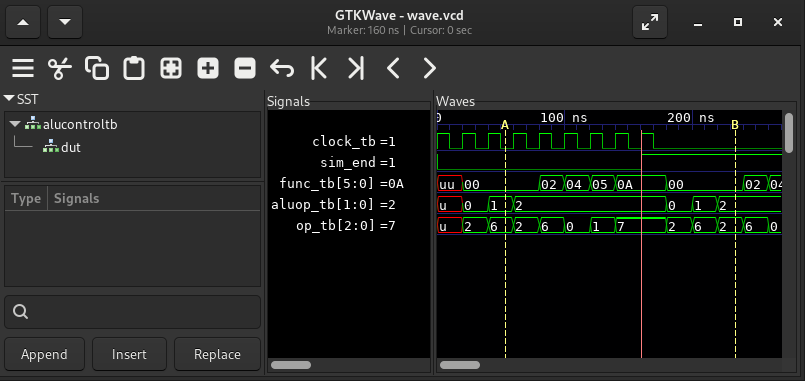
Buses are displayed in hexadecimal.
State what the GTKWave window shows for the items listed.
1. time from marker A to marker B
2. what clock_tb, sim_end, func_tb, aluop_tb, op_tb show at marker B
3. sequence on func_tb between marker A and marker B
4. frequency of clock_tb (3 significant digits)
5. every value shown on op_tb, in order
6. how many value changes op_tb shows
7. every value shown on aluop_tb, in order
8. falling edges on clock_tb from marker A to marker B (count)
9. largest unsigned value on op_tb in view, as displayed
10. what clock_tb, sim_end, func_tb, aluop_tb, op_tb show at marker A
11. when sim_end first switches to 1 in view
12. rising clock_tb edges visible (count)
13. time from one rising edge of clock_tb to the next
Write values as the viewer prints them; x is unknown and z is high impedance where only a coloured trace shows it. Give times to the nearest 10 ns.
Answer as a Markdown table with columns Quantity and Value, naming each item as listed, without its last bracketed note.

| Quantity | Value |
|---|---|
| time from marker A to marker B | 180 ns |
| what clock_tb, sim_end, func_tb, aluop_tb, op_tb show at marker B | clock_tb=0, sim_end=1, func_tb=00, aluop_tb=2, op_tb=2 |
| sequence on func_tb between marker A and marker B | 00, 02, 04, 05, 0A, 00 |
| frequency of clock_tb | 50.0 MHz |
| every value shown on op_tb, in order | u, 2, 6, 2, 6, 0, 1, 7, 2, 6, 2, 6, 0 |
| how many value changes op_tb shows | 12 |
| every value shown on aluop_tb, in order | u, 0, 1, 2, 0, 1, 2 |
| falling edges on clock_tb from marker A to marker B | 6 |
| largest unsigned value on op_tb in view, as displayed | 7 |
| what clock_tb, sim_end, func_tb, aluop_tb, op_tb show at marker A | clock_tb=0, sim_end=0, func_tb=00, aluop_tb=1, op_tb=6 |
| when sim_end first switches to 1 in view | 160 ns |
| rising clock_tb edges visible | 8 |
| time from one rising edge of clock_tb to the next | 20 ns |
